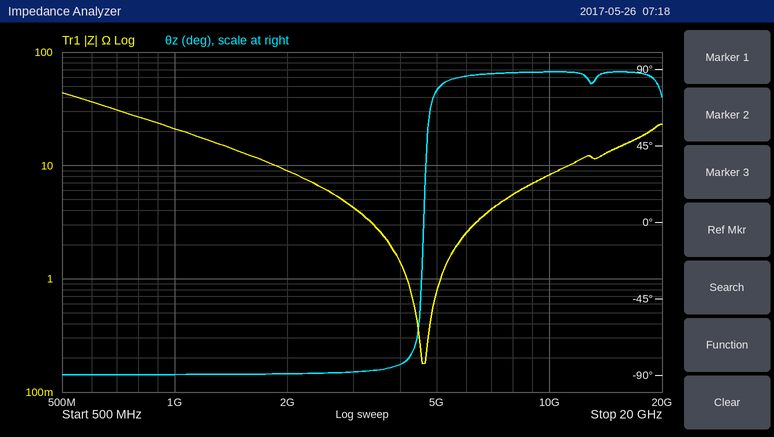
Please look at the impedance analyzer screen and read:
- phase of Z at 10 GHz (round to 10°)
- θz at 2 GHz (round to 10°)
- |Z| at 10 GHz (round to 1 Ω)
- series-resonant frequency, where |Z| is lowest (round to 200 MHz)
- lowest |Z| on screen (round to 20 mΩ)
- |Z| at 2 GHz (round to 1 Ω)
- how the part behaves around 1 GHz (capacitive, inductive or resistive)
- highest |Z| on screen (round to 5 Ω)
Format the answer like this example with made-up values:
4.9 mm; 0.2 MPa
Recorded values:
90°; -90°; 8 Ω; 4.6 GHz; 180 mΩ; 9 Ω; capacitive; 45 Ω
